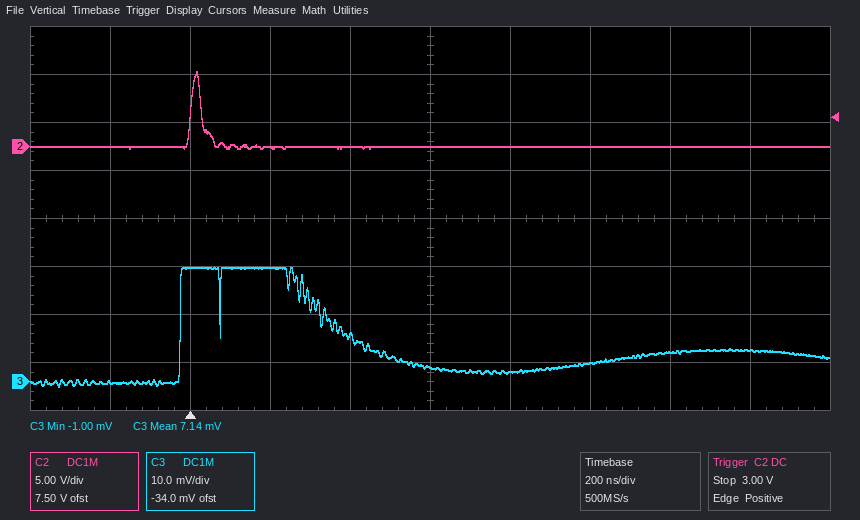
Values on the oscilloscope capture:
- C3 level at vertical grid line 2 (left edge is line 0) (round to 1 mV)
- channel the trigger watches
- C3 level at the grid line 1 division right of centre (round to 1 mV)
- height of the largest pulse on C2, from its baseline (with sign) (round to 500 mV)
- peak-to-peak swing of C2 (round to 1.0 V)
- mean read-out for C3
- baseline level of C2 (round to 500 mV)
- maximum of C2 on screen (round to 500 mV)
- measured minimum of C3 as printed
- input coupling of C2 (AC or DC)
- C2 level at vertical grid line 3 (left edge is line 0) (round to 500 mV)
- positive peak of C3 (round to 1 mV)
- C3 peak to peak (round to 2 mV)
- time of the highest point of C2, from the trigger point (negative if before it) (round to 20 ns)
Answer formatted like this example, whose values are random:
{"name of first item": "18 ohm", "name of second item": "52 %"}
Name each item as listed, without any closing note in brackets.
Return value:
{"C3 level at vertical grid line 2 (left edge is line 0)": "24 mV", "channel the trigger watches": "C2", "C3 level at the grid line 1 division right of centre": "2 mV", "height of the largest pulse on C2, from its baseline (with sign)": "+8.0 V", "peak-to-peak swing of C2": "8.0 V", "mean read-out for C3": "7.14 mV", "baseline level of C2": "0.0 V", "maximum of C2 on screen": "8.0 V", "measured minimum of C3 as printed": "-1.00 mV", "input coupling of C2": "DC", "C2 level at vertical grid line 3 (left edge is line 0)": "0.0 V", "positive peak of C3": "24 mV", "C3 peak to peak": "24 mV", "time of the highest point of C2, from the trigger point (negative if before it)": "+20 ns"}
